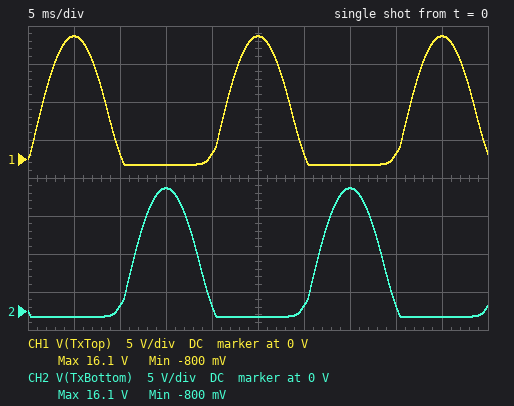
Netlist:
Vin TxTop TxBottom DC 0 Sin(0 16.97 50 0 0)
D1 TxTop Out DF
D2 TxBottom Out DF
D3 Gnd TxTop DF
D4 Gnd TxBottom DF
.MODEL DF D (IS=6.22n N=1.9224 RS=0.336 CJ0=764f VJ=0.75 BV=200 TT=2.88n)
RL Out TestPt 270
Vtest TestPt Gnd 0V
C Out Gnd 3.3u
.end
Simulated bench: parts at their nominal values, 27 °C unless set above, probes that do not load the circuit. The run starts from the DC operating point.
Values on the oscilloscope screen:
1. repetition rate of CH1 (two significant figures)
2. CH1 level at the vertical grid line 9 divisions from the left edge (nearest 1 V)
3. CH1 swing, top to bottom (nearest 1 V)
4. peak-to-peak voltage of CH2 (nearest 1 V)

50 Hz
16 V
17 V
17 V
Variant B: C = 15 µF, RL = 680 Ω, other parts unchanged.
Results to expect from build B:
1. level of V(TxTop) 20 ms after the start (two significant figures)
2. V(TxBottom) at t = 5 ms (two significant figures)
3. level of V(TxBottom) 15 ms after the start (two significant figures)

5.0 V
-760 mV
16 V
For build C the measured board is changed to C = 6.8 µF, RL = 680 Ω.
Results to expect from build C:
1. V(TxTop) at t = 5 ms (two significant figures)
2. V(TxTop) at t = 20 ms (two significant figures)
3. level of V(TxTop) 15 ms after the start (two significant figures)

16 V
3.3 V
-760 mV
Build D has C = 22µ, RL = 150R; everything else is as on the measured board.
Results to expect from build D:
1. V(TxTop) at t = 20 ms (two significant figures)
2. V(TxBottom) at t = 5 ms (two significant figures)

2.5 V
-860 mV
